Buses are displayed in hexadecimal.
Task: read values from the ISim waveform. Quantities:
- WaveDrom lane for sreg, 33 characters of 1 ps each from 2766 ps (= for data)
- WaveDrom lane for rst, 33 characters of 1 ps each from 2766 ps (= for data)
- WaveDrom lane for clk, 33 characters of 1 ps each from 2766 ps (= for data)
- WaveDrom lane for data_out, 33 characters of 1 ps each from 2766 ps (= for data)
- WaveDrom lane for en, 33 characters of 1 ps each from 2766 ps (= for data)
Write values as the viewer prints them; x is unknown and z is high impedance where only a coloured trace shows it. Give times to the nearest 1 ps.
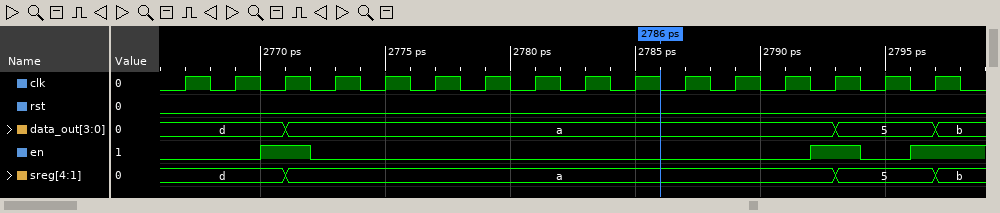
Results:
{name: 'sreg', wave: '=....=.....................=...=.', data: 'd a 5 b'}
{name: 'rst', wave: '0................................'}
{name: 'clk', wave: '010101010101010101010101010101010'}
{name: 'data_out', wave: '=....=.....................=...=.', data: 'd a 5 b'}
{name: 'en', wave: '0...1.0...................1.0.1..'}
